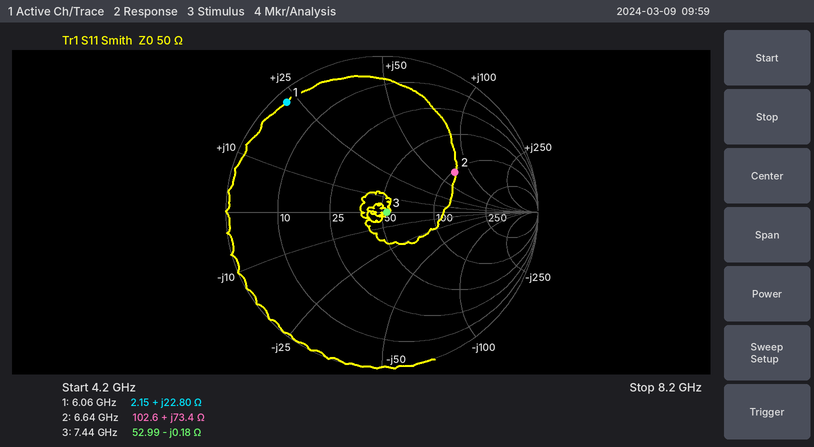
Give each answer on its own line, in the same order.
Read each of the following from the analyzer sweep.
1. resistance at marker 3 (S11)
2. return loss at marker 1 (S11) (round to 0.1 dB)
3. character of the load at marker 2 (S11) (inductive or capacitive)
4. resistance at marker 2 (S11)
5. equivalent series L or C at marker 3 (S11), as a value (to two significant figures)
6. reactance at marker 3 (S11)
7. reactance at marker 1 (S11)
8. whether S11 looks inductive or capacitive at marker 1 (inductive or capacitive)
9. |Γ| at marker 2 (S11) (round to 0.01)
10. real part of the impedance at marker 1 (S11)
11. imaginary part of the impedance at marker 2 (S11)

52.99 Ω
0.6 dB
inductive
102.6 Ω
120 pF
-0.18 Ω
+22.80 Ω
inductive
0.53
2.15 Ω
+73.4 Ω
